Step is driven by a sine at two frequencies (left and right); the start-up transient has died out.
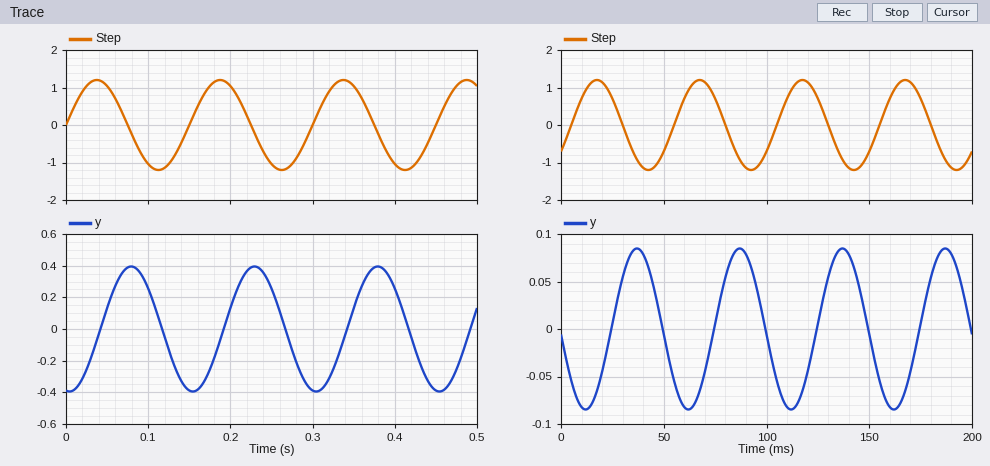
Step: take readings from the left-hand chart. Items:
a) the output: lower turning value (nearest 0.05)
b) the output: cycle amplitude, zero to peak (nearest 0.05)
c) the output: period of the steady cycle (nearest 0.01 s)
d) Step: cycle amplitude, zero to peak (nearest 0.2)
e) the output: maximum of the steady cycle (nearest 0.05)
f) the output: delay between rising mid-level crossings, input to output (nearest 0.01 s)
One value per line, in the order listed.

-0.40
0.40
0.15 s
1.2
0.40
0.04 s
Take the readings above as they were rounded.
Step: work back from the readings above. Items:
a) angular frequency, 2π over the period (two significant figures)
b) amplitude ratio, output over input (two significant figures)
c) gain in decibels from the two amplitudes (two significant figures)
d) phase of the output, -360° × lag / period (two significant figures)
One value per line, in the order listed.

42 rad/s
0.33
-9.5 dB
-96°
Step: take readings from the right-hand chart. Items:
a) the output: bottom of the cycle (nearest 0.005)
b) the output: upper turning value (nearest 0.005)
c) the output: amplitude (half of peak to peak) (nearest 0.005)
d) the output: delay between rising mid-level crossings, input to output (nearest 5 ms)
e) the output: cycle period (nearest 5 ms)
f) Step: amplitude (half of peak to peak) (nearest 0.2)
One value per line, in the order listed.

-0.085
0.085
0.085
20 ms
50 ms
1.2
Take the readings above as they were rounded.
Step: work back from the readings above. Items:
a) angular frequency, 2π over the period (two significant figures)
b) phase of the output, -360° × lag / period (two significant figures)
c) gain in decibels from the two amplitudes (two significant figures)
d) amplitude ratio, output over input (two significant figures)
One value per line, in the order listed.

0.13 rad/ms
-140°
-23 dB
0.071
